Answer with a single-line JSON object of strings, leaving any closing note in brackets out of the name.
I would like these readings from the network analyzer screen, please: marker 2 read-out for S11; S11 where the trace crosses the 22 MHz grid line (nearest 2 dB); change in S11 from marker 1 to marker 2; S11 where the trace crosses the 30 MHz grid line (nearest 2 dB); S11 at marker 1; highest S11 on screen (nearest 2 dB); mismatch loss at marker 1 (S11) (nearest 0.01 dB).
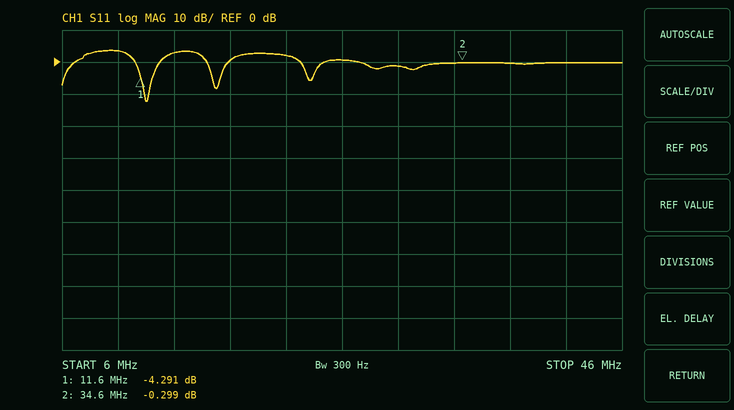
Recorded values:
{"marker 2 read-out for S11": "-0.299 dB", "S11 where the trace crosses the 22 MHz grid line": "2 dB", "change in S11 from marker 1 to marker 2": "3.992 dB", "S11 where the trace crosses the 30 MHz grid line": "-2 dB", "S11 at marker 1": "-4.291 dB", "highest S11 on screen": "4 dB", "mismatch loss at marker 1 (S11)": "2.02 dB"}
